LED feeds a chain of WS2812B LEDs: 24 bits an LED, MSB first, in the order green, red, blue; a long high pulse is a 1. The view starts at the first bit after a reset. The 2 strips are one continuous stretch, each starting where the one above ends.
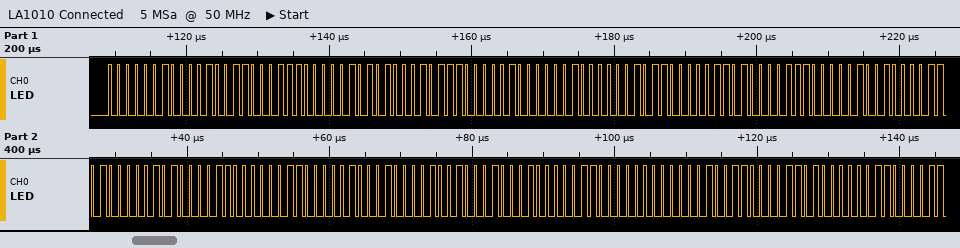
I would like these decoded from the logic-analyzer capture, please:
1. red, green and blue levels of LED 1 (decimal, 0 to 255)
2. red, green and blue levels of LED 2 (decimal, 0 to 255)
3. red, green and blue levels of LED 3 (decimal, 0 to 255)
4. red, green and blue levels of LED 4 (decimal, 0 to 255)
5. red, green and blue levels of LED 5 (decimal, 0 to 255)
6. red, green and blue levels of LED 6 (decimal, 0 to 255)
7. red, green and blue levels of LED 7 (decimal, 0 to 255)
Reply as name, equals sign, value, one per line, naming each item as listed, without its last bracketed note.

red, green and blue levels of LED 1 = 19, 2, 28
red, green and blue levels of LED 2 = 23, 21, 4
red, green and blue levels of LED 3 = 22, 8, 13
red, green and blue levels of LED 4 = 9, 14, 13
red, green and blue levels of LED 5 = 12, 5, 12
red, green and blue levels of LED 6 = 9, 17, 17
red, green and blue levels of LED 7 = 0, 6, 19
